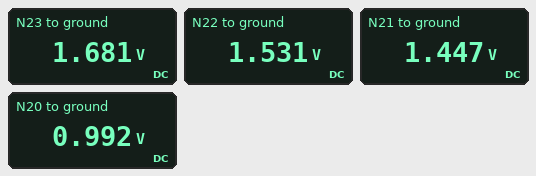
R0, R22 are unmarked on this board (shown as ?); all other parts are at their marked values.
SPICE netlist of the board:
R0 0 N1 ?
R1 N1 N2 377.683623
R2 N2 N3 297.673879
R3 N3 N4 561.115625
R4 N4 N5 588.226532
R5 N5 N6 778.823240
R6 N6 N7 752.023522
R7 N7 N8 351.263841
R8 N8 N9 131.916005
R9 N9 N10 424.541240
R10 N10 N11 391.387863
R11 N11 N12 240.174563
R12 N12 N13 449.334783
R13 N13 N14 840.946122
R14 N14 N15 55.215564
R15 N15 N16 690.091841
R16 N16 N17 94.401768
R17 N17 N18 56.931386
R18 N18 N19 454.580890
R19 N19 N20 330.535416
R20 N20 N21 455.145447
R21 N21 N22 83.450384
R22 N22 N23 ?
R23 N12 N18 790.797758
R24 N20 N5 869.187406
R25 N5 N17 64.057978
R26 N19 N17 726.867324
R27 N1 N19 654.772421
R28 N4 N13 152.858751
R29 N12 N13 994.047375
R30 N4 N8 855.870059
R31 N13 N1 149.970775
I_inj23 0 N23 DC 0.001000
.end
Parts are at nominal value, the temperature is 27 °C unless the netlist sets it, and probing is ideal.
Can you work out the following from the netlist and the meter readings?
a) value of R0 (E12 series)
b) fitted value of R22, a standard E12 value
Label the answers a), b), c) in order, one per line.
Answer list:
a) 470 Ω
b) 150 Ω
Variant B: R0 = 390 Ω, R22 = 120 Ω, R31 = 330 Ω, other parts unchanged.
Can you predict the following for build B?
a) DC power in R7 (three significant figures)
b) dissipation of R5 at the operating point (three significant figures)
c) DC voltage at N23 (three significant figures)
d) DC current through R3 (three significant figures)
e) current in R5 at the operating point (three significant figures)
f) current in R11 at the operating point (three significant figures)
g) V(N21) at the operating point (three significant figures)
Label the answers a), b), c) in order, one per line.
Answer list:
a) 930 nW
b) 2.06 µW
c) 1.60 V
d) 119 µA
e) 51.5 µA
f) 10.6 µA
g) 1.40 V
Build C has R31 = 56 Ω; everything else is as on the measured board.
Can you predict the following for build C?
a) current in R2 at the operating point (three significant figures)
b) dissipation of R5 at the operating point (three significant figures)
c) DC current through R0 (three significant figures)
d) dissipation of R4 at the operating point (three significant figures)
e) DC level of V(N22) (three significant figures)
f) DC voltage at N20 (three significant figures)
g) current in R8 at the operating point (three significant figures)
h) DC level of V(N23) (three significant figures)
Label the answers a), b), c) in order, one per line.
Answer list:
a) 53.1 µA
b) 2.65 µW
c) 1.00 mA
d) 36.4 µW
e) 1.51 V
f) 970 mV
g) 15.7 µA
h) 1.66 V
